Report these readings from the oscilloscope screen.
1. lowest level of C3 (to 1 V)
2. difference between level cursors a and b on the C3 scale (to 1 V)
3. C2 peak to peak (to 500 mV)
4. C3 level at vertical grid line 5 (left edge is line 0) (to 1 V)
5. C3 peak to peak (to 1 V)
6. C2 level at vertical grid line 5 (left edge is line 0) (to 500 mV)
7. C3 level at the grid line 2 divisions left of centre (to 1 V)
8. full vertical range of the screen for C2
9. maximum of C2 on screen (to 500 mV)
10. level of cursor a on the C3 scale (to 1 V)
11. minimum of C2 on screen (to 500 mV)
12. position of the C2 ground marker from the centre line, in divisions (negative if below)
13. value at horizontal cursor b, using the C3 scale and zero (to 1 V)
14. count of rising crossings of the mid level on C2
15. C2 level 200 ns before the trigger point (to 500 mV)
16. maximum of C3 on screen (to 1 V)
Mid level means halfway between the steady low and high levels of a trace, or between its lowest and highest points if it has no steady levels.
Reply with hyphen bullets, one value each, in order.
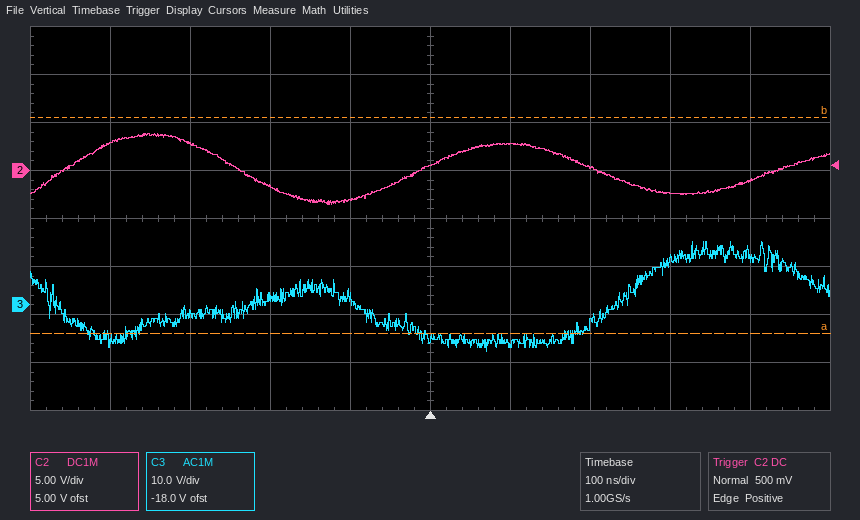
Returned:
- -10 V
- 45 V
- 7.5 V
- -7 V
- 23 V
- 500 mV
- 2 V
- 40 V
- 4.0 V
- -6 V
- -3.5 V
- +1.0 div
- 39 V
- 3
- -1.5 V
- 13 V
